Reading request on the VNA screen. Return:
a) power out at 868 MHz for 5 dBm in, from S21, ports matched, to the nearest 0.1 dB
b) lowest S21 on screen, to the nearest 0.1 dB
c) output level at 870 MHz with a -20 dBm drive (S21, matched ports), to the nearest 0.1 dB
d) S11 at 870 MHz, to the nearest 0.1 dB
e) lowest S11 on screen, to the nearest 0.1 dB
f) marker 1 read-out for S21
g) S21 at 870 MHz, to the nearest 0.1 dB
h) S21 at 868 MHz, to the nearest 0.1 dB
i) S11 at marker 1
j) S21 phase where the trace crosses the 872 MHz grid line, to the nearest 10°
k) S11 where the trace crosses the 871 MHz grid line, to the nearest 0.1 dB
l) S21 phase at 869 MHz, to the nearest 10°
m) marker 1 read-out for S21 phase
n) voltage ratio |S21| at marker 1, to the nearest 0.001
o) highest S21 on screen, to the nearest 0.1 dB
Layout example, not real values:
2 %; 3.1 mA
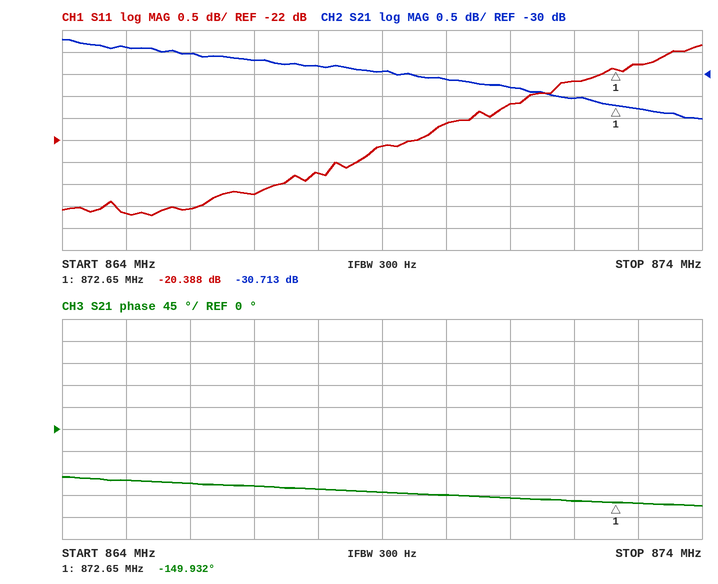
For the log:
-24.8 dBm; -31.0 dB; -50.1 dBm; -21.6 dB; -23.7 dB; -30.713 dB; -30.1 dB; -29.8 dB; -20.388 dB; -150°; -21.2 dB; -130°; -149.932°; 0.029; -29.2 dB
